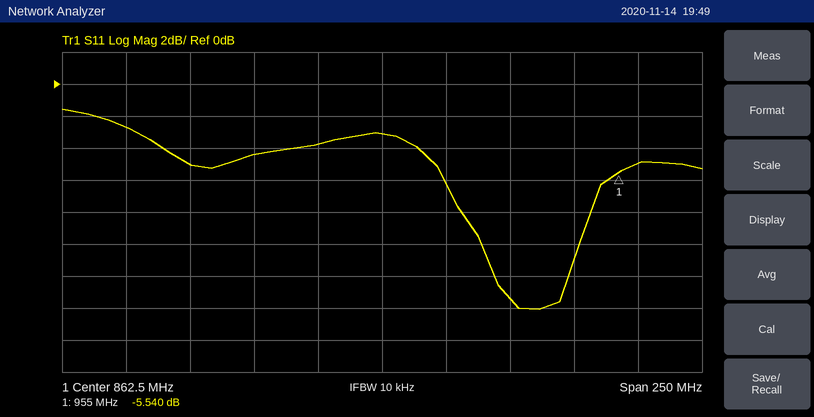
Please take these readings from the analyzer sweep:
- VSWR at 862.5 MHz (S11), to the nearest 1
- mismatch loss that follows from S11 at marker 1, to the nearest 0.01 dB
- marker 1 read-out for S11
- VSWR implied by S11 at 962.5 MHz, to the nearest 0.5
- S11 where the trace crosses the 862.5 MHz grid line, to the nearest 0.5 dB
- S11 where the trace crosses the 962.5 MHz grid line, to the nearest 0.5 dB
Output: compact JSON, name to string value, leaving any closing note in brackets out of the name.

{"VSWR at 862.5 MHz (S11), to the nearest 1": "6", "mismatch loss that follows from S11 at marker 1, to the nearest 0.01 dB": "1.42 dB", "marker 1 read-out for S11": "-5.540 dB", "VSWR implied by S11 at 962.5 MHz, to the nearest 0.5": "3.5", "S11 where the trace crosses the 862.5 MHz grid line, to the nearest 0.5 dB": "-3.0 dB", "S11 where the trace crosses the 962.5 MHz grid line, to the nearest 0.5 dB": "-5.0 dB"}
